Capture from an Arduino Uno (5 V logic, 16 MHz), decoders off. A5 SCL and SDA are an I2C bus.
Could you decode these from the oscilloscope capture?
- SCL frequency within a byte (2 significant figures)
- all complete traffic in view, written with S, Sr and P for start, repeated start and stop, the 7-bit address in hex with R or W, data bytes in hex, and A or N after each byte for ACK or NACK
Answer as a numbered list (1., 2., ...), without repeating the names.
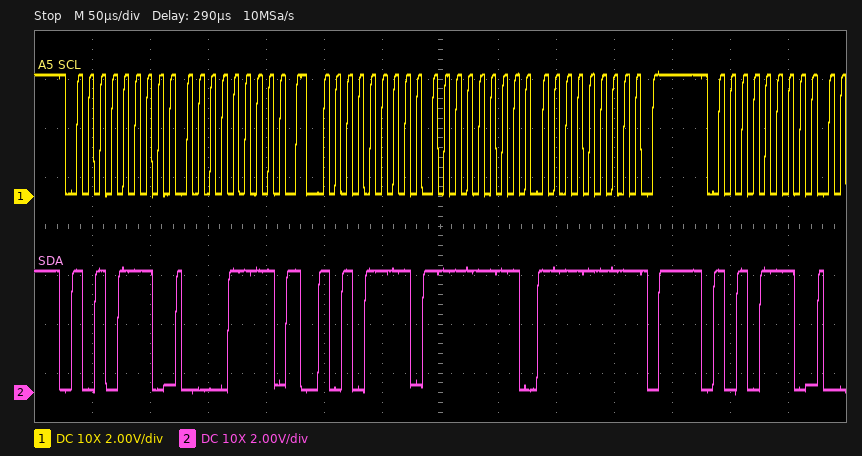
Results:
1. 100 kHz
2. S 57W A 0F A Sr 57R A FF A FF N P S 57W A
